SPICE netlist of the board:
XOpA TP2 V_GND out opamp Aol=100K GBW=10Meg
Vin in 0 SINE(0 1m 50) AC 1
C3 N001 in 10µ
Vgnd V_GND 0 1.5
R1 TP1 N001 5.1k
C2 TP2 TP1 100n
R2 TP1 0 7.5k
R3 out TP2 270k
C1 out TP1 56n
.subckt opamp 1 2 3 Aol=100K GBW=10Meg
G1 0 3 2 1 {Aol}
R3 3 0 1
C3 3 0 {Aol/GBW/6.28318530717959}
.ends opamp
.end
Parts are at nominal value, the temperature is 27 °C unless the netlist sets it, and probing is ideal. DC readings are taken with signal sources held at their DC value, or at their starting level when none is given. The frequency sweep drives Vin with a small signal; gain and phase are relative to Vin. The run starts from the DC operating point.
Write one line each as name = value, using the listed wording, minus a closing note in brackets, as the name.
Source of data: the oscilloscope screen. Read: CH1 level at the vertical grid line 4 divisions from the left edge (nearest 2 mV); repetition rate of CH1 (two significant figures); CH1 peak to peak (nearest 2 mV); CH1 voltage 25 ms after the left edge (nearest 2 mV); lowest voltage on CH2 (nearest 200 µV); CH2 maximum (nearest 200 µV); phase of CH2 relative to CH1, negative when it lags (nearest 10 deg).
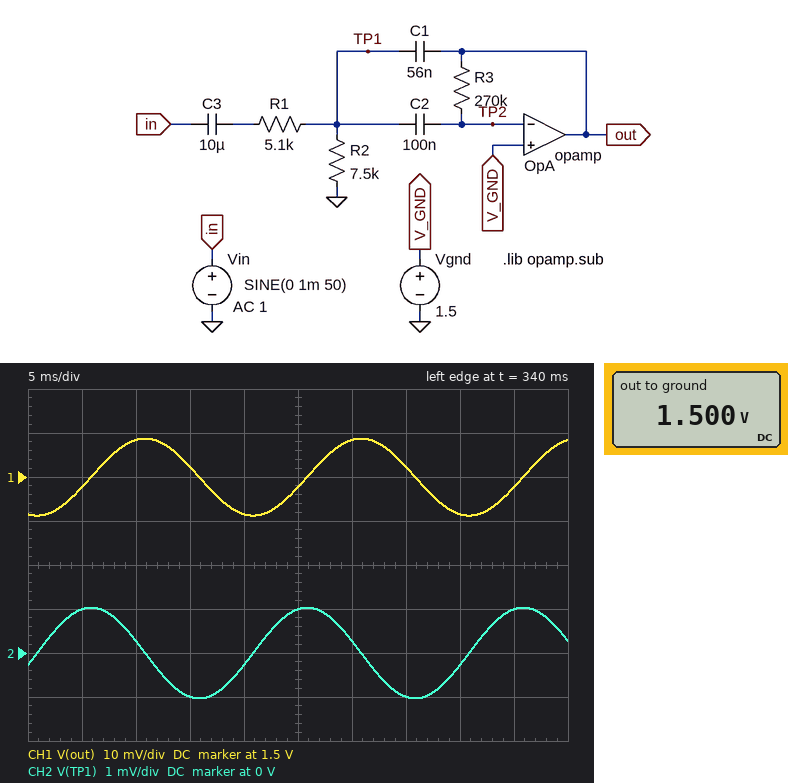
CH1 level at the vertical grid line 4 divisions from the left edge = 1.492 V
repetition rate of CH1 = 50 Hz
CH1 peak to peak = 18 mV
CH1 voltage 25 ms after the left edge = 1.498 V
lowest voltage on CH2 = -1.0 mV
CH2 maximum = 1.0 mV
phase of CH2 relative to CH1, negative when it lags = 90 deg
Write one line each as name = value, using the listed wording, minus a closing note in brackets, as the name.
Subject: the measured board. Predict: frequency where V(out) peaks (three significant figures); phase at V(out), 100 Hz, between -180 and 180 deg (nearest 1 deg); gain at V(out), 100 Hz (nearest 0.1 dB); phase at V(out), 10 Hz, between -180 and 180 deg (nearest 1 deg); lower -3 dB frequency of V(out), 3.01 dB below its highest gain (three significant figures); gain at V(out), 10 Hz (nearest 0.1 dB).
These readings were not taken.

frequency where V(out) peaks = 74.5 Hz
phase at V(out), 100 Hz, between -180 and 180 deg = 113 deg
gain at V(out), 100 Hz = 21.3 dB
phase at V(out), 10 Hz, between -180 and 180 deg = -85 deg
lower -3 dB frequency of V(out), 3.01 dB below its highest gain = 65.9 Hz
gain at V(out), 10 Hz = 0.1 dB
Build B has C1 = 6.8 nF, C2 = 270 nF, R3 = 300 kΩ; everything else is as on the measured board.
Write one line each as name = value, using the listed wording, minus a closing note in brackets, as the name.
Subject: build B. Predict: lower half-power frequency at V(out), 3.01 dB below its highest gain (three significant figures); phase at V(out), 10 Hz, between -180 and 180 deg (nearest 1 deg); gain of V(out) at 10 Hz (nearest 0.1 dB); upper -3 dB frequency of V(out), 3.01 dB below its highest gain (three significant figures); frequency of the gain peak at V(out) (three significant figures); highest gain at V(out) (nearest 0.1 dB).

lower half-power frequency at V(out), 3.01 dB below its highest gain = 89.3 Hz
phase at V(out), 10 Hz, between -180 and 180 deg = -86 deg
gain of V(out) at 10 Hz = 9.5 dB
upper -3 dB frequency of V(out), 3.01 dB below its highest gain = 171 Hz
frequency of the gain peak at V(out) = 124 Hz
highest gain at V(out) = 35.0 dB
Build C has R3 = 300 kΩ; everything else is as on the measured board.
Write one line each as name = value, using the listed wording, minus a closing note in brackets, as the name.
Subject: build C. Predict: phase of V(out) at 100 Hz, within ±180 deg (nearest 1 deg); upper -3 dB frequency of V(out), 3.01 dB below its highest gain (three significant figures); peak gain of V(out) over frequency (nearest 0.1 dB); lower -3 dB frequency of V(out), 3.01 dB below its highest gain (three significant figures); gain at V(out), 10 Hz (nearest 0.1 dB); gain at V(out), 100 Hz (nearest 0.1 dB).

phase of V(out) at 100 Hz, within ±180 deg = 109 deg
upper -3 dB frequency of V(out), 3.01 dB below its highest gain = 79.5 Hz
peak gain of V(out) over frequency = 30.5 dB
lower -3 dB frequency of V(out), 3.01 dB below its highest gain = 62.8 Hz
gain at V(out), 10 Hz = 1.1 dB
gain at V(out), 100 Hz = 20.5 dB
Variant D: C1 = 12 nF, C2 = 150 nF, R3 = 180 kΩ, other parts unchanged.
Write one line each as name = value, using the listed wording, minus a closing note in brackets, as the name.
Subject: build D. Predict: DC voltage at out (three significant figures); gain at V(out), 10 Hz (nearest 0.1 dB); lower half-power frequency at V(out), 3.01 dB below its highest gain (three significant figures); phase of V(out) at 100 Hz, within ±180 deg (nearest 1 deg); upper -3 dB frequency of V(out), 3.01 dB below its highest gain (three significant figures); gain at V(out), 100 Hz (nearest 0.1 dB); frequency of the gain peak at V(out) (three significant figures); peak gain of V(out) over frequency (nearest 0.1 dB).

DC voltage at out = 1.50 V
gain at V(out), 10 Hz = 0 dB
lower half-power frequency at V(out), 3.01 dB below its highest gain = 125 Hz
phase of V(out) at 100 Hz, within ±180 deg = -116 deg
upper -3 dB frequency of V(out), 3.01 dB below its highest gain = 207 Hz
gain at V(out), 100 Hz = 23.3 dB
frequency of the gain peak at V(out) = 161 Hz
peak gain of V(out) over frequency = 30.1 dB
